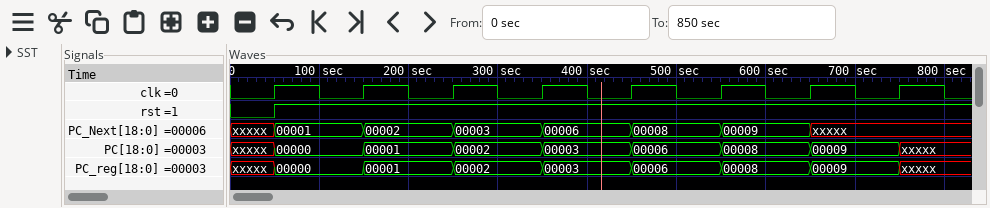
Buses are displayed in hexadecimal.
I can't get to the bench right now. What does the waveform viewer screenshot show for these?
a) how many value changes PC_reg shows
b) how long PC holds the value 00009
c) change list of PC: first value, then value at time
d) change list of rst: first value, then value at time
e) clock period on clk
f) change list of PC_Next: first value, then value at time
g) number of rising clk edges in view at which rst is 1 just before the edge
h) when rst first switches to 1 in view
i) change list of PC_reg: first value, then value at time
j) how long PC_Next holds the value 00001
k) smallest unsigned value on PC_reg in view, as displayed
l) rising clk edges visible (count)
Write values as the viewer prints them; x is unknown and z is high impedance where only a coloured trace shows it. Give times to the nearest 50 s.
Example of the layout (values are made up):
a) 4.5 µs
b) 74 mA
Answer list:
a) 8
b) 100 s
c) xxxxx, 00000 at 50 s, 00001 at 150 s, 00002 at 250 s, 00003 at 350 s, 00006 at 450 s, 00008 at 550 s, 00009 at 650 s, xxxxx at 750 s
d) 0, 1 at 50 s
e) 100 s
f) xxxxx, 00001 at 50 s, 00002 at 150 s, 00003 at 250 s, 00006 at 350 s, 00008 at 450 s, 00009 at 550 s, xxxxx at 650 s
g) 7
h) 50 s
i) xxxxx, 00000 at 50 s, 00001 at 150 s, 00002 at 250 s, 00003 at 350 s, 00006 at 450 s, 00008 at 550 s, 00009 at 650 s, xxxxx at 750 s
j) 100 s
k) 00000
l) 8
